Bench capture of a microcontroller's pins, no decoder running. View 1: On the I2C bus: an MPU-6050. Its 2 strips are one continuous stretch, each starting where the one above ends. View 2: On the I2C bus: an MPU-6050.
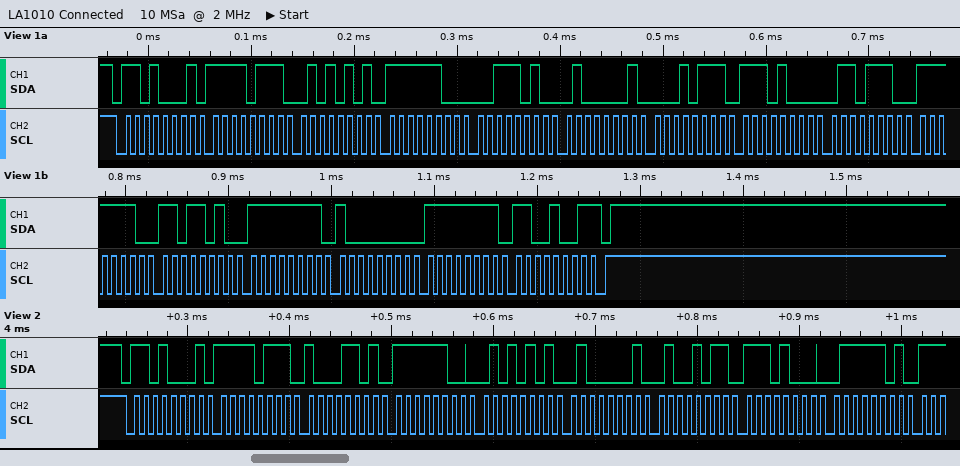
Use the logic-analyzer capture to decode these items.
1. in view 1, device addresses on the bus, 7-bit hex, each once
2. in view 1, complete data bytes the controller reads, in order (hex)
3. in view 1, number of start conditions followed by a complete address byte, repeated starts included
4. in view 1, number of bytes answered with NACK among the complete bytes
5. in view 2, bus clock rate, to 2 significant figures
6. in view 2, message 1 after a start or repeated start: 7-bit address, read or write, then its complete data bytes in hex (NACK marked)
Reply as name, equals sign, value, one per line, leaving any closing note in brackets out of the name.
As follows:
in view 1, device addresses on the bus, 7-bit hex, each once = 0x68
in view 1, complete data bytes the controller reads, in order = F7 55 FC 3A 41 17 E8 6E FE DA FF 80 FF C9
in view 1, number of start conditions followed by a complete address byte, repeated starts included = 1
in view 1, number of bytes answered with NACK among the complete bytes = 1
in view 2, bus clock rate, to 2 significant figures = 110 kHz
in view 2, message 1 after a start or repeated start: 7-bit address, read or write, then its complete data bytes in hex = 0x68 read: F7 8D FC 55 41 4B E8 7D
